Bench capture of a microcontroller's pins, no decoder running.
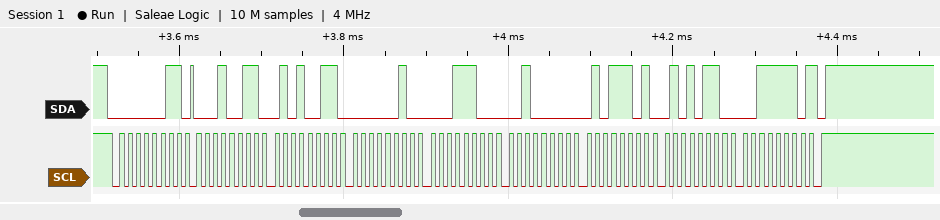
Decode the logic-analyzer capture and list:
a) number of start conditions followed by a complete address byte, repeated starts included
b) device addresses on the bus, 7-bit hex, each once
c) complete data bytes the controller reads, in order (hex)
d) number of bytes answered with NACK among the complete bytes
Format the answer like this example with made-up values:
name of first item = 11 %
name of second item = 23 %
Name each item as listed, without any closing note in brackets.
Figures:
number of start conditions followed by a complete address byte, repeated starts included = 1
device addresses on the bus, 7-bit hex, each once = 0x01
complete data bytes the controller reads, in order = 13 53 02 1C 20 5D 56 3E
number of bytes answered with NACK among the complete bytes = 1
